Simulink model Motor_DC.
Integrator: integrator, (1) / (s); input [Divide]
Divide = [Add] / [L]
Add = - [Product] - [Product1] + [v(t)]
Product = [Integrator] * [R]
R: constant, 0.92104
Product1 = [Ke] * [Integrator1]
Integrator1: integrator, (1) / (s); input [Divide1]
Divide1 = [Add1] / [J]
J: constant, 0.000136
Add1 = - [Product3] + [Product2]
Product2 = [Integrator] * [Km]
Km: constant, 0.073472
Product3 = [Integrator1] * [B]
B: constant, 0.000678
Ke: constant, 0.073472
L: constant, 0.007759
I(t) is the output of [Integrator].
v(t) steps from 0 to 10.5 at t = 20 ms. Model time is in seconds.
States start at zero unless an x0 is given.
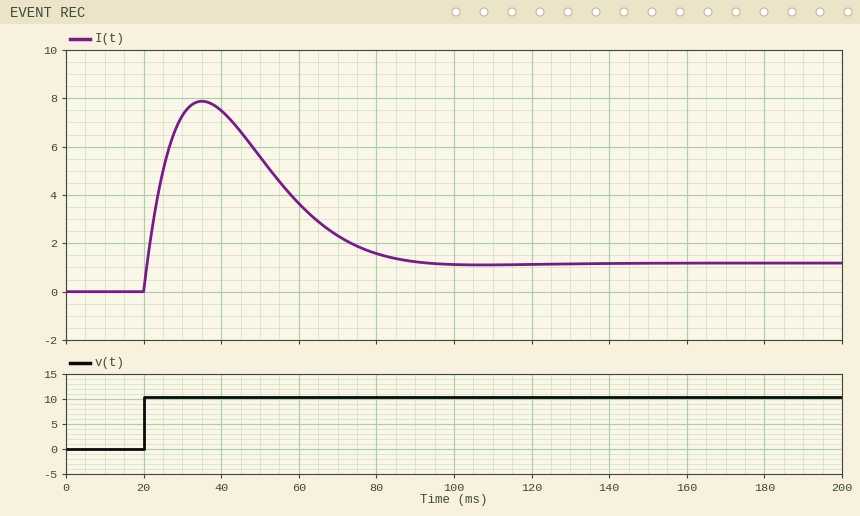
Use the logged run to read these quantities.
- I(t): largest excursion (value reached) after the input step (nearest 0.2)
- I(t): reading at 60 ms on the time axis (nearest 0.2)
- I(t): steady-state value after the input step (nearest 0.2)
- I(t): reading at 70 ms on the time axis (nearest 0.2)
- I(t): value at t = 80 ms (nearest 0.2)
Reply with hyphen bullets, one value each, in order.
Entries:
- 7.8
- 3.6
- 1.2
- 2.4
- 1.6
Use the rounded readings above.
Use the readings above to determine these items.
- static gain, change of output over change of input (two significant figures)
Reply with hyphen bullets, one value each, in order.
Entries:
- 0.11
